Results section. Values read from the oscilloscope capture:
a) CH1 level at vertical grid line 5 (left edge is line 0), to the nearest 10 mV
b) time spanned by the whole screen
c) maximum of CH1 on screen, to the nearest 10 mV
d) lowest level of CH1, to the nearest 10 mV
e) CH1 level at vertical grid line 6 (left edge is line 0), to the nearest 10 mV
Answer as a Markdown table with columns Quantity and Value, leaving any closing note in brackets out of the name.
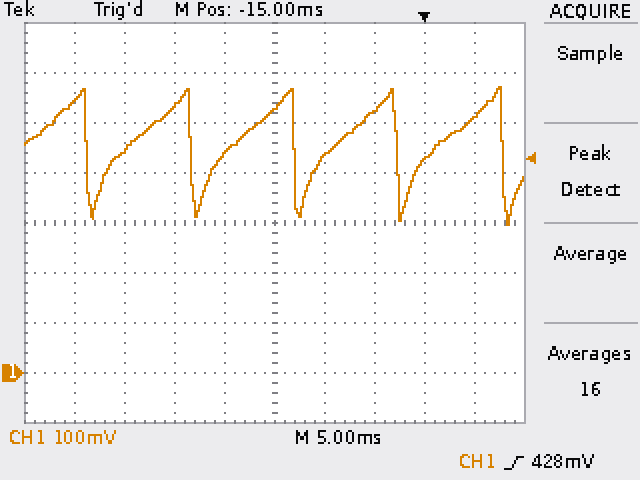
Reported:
| Quantity | Value |
|---|---|
| CH1 level at vertical grid line 5 (left edge is line 0), to the nearest 10 mV | 530 mV |
| time spanned by the whole screen | 50 ms |
| maximum of CH1 on screen, to the nearest 10 mV | 570 mV |
| lowest level of CH1, to the nearest 10 mV | 300 mV |
| CH1 level at vertical grid line 6 (left edge is line 0), to the nearest 10 mV | 430 mV |
